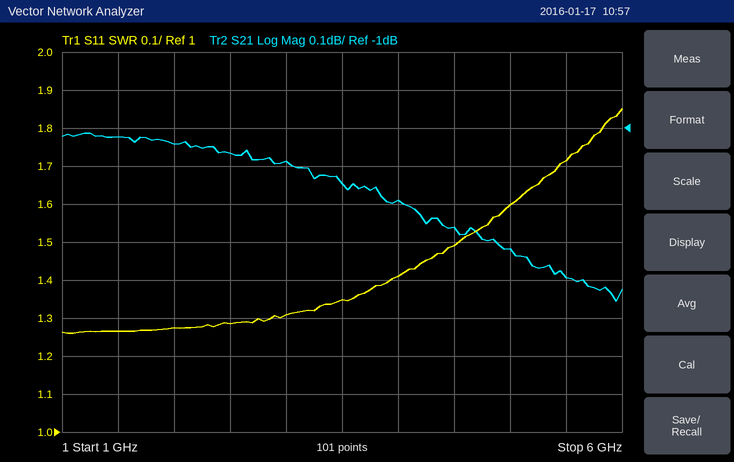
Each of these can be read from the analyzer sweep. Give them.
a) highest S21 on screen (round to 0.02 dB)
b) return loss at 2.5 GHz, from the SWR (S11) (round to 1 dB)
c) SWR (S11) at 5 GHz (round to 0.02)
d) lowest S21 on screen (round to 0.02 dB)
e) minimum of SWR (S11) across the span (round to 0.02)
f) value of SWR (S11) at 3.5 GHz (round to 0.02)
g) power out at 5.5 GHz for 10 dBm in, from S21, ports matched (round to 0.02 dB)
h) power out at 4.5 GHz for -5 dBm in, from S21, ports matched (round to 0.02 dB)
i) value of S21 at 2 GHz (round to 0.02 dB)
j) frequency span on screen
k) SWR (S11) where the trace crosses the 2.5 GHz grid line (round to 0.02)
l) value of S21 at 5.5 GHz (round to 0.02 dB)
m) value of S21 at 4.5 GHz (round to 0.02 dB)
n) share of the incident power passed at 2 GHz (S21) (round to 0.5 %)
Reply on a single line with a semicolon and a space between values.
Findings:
-1.02 dB; 18 dB; 1.60; -1.46 dB; 1.26; 1.34; 8.60 dBm; -6.26 dBm; -1.04 dB; 5 GHz; 1.28; -1.40 dB; -1.26 dB; 78.5 %
